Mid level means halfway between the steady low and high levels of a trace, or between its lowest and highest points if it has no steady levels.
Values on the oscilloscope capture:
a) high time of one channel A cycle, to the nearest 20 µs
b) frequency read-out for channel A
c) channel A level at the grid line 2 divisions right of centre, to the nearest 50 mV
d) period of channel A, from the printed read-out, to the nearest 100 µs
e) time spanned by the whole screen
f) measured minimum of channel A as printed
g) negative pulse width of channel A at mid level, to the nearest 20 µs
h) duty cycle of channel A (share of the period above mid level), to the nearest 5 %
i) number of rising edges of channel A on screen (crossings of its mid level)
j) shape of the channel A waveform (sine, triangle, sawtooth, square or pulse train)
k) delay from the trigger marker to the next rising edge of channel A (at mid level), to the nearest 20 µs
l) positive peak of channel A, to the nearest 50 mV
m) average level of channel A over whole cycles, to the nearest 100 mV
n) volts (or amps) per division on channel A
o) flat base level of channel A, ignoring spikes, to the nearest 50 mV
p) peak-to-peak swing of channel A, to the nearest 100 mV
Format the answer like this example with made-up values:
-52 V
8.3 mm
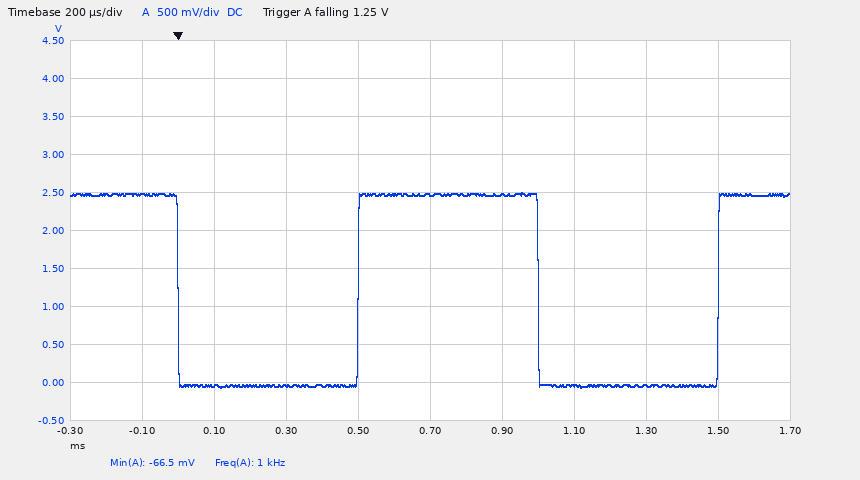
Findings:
500 µs
1 kHz
-50 mV
1.0 ms
2 ms
-66.5 mV
500 µs
50 %
2
square
500 µs
2.50 V
1.2 V
500 mV
-50 mV
2.60 V
